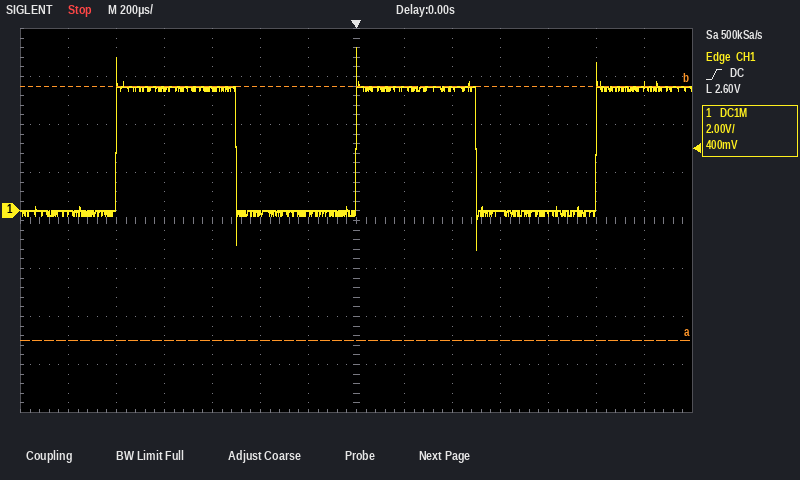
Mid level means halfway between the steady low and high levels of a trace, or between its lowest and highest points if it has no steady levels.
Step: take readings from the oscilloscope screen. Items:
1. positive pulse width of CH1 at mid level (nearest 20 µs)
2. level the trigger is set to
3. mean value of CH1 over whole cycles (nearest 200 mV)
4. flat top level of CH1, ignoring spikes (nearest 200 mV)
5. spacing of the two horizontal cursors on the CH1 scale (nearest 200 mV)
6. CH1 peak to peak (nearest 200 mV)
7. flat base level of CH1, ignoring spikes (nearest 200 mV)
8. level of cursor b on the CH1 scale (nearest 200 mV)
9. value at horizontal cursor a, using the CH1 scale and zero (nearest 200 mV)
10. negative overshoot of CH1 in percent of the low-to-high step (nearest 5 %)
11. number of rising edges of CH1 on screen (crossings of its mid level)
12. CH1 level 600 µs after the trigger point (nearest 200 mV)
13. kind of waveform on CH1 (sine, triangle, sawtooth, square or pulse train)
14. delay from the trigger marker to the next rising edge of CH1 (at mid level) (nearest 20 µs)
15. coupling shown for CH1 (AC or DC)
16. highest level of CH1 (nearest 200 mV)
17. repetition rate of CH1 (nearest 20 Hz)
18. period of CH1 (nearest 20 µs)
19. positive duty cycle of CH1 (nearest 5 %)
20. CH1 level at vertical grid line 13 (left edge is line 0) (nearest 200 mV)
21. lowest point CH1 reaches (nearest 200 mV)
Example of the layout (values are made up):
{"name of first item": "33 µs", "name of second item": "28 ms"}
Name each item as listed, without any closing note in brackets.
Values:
{"positive pulse width of CH1 at mid level": "500 µs", "level the trigger is set to": "2.60 V", "mean value of CH1 over whole cycles": "2.6 V", "flat top level of CH1, ignoring spikes": "5.2 V", "spacing of the two horizontal cursors on the CH1 scale": "10.6 V", "CH1 peak to peak": "8.4 V", "flat base level of CH1, ignoring spikes": "0.0 V", "level of cursor b on the CH1 scale": "5.2 V", "value at horizontal cursor a, using the CH1 scale and zero": "-5.4 V", "negative overshoot of CH1 in percent of the low-to-high step": "30 %", "number of rising edges of CH1 on screen": "3", "CH1 level 600 µs after the trigger point": "0.0 V", "kind of waveform on CH1": "square", "delay from the trigger marker to the next rising edge of CH1 (at mid level)": "1.00 ms", "coupling shown for CH1": "DC", "highest level of CH1": "6.8 V", "repetition rate of CH1": "1.00 kHz", "period of CH1": "1.00 ms", "positive duty cycle of CH1": "50 %", "CH1 level at vertical grid line 13 (left edge is line 0)": "5.2 V", "lowest point CH1 reaches": "-1.6 V"}
